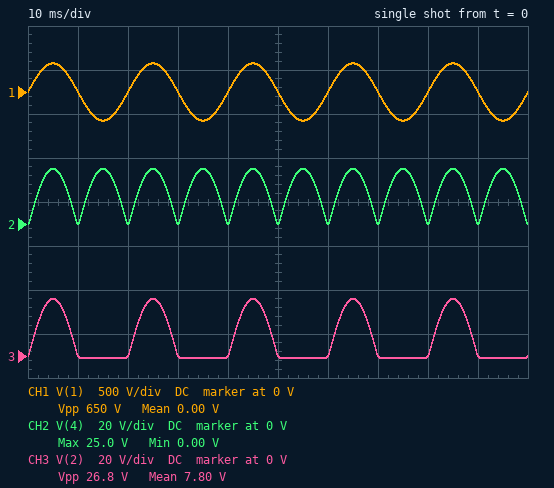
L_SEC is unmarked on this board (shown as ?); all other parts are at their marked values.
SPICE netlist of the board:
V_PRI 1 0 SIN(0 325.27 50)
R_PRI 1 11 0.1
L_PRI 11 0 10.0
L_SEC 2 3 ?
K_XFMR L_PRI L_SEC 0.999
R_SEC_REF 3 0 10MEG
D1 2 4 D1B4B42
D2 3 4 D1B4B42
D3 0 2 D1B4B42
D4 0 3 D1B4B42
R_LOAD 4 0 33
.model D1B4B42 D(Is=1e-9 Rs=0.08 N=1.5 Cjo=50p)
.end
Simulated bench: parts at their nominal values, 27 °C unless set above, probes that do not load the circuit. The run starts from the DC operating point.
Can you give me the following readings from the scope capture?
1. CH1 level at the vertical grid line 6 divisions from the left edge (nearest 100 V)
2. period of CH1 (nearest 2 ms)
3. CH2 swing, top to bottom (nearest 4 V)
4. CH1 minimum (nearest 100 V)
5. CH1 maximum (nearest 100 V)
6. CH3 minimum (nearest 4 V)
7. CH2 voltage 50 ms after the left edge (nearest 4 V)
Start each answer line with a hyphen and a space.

- 0 V
- 20 ms
- 24 V
- -300 V
- 300 V
- 0 V
- 0 V
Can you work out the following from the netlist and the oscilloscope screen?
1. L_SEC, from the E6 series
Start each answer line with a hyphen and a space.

- 68 mH
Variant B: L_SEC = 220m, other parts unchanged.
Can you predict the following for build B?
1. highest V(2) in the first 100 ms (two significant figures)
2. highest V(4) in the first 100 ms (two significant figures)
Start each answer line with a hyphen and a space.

- 47 V
- 46 V
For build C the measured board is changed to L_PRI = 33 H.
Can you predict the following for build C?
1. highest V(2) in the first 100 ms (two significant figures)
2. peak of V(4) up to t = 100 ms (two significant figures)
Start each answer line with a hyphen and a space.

- 14 V
- 13 V
